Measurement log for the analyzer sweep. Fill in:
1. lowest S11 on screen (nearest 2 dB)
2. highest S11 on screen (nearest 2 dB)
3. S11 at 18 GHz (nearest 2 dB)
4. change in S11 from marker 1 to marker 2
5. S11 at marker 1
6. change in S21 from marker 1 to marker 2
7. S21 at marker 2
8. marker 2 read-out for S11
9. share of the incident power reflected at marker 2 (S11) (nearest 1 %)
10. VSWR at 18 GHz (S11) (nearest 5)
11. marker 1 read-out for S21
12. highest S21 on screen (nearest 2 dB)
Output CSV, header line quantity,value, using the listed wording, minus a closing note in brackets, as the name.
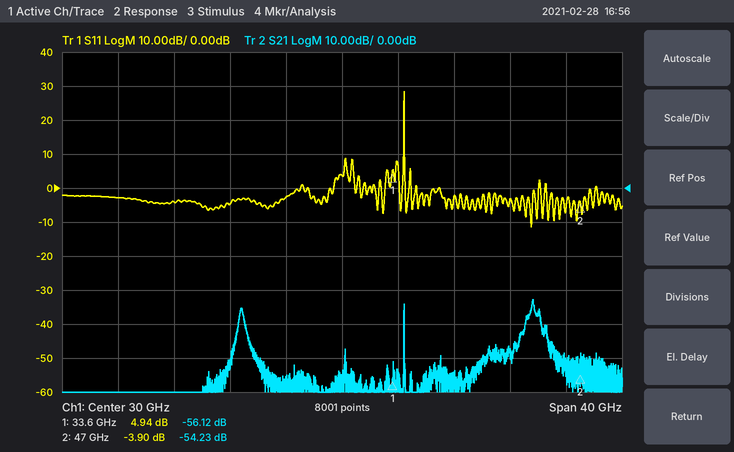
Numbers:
quantity,value
lowest S11 on screen,-12 dB
highest S11 on screen,28 dB
S11 at 18 GHz,-4 dB
change in S11 from marker 1 to marker 2,-8.84 dB
S11 at marker 1,4.94 dB
change in S21 from marker 1 to marker 2,1.89 dB
S21 at marker 2,-54.23 dB
marker 2 read-out for S11,-3.90 dB
share of the incident power reflected at marker 2 (S11),41 %
VSWR at 18 GHz (S11),5
marker 1 read-out for S21,-56.12 dB
highest S21 on screen,-32 dB
